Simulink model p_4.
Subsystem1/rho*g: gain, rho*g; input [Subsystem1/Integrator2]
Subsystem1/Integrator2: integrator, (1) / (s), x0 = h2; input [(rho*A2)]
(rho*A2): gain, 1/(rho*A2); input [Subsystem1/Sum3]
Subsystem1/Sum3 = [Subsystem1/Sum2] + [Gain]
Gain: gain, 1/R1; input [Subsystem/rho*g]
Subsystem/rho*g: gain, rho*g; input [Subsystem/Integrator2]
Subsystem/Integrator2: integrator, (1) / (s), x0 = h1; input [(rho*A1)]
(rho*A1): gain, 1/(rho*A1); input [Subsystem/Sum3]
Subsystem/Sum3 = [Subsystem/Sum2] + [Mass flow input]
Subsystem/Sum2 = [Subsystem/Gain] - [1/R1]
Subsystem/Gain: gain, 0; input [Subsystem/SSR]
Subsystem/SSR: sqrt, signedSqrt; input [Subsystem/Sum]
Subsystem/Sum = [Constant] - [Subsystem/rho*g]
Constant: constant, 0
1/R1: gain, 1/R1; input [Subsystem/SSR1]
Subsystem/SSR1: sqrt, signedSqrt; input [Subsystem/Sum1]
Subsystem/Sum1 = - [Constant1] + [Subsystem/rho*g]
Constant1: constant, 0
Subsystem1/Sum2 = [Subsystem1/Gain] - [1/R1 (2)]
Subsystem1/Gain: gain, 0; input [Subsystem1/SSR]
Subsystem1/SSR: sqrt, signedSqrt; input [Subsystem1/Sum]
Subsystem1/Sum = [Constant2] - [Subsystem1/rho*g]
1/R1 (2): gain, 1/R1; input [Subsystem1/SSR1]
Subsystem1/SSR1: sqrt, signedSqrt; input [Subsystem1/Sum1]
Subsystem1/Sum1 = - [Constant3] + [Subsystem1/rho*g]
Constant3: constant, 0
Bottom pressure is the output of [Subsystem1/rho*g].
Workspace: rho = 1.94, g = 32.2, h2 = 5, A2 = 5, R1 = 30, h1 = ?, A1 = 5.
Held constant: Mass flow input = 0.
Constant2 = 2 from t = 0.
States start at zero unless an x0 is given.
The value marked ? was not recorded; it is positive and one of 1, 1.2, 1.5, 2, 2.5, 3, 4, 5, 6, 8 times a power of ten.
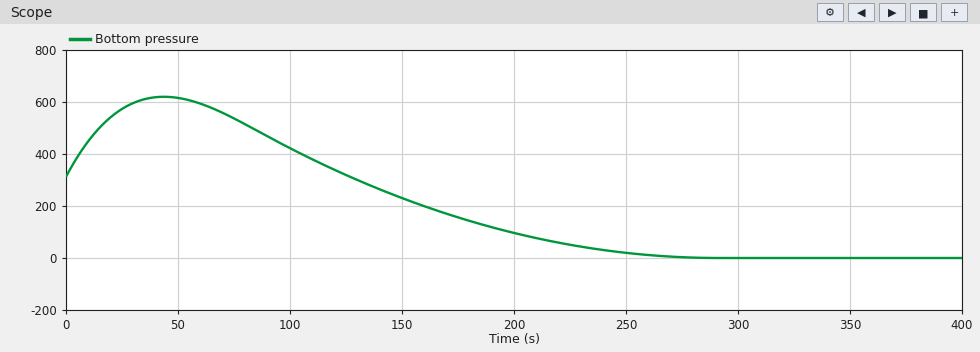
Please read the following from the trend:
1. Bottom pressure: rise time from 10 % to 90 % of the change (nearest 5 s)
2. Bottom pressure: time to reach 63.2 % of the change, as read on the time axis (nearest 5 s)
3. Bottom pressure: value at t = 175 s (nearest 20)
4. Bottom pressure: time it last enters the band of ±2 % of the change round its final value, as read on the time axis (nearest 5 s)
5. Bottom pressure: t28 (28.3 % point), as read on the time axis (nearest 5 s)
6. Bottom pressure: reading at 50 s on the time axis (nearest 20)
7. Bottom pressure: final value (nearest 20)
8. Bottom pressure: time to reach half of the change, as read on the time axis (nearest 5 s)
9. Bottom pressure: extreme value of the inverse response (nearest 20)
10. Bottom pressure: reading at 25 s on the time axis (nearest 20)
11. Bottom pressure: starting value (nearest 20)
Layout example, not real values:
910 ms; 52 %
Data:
105 s; 190 s; 160; 270 s; 150 s; 620; 0; 175 s; 620; 580; 320
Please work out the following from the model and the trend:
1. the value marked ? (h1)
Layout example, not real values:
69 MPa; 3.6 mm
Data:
1.5
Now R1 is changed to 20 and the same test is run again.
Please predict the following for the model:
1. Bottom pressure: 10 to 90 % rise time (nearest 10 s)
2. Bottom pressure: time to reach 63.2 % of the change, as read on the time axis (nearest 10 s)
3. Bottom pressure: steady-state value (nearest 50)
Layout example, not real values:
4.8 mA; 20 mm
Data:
70 s; 130 s; 0
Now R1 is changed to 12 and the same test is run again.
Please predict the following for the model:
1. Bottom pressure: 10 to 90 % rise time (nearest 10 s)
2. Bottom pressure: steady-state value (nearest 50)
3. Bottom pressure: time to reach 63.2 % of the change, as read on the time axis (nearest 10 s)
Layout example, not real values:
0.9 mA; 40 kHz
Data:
40 s; 0; 80 s
